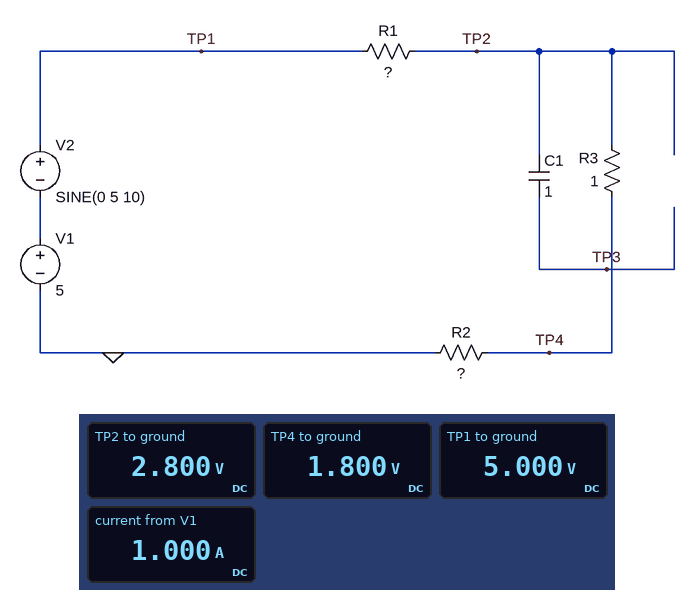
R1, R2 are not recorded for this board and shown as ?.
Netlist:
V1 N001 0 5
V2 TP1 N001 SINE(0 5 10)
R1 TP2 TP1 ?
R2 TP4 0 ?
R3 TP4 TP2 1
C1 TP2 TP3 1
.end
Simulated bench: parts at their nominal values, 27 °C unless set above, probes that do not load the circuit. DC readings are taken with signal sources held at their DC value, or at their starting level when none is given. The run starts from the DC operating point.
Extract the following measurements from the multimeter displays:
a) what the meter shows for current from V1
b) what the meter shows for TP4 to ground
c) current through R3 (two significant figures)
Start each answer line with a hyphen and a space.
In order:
- 1.000 A
- 1.800 V
- 1.0 A
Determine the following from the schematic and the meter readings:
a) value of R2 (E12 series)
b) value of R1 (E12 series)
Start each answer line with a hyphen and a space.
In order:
- 1.8 Ω
- 2.2 Ω
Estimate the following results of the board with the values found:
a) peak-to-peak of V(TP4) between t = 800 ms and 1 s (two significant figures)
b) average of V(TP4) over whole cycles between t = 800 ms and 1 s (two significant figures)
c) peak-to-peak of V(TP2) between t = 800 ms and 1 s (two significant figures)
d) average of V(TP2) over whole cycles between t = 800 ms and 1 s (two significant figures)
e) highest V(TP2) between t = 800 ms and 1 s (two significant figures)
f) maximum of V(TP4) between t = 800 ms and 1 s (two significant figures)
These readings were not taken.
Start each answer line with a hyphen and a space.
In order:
- 3.6 V
- 1.8 V
- 5.6 V
- 2.8 V
- 5.6 V
- 3.6 V
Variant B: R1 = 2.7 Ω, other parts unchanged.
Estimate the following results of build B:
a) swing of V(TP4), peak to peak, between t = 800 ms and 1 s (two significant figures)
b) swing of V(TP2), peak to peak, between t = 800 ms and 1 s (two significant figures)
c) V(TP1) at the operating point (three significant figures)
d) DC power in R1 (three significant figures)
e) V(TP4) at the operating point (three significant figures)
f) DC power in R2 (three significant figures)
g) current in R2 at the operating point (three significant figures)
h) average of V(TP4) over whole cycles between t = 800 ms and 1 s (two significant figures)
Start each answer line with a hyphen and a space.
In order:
- 3.3 V
- 5.1 V
- 5.00 V
- 2.23 W
- 1.64 V
- 1.49 W
- 909 mA
- 1.6 V
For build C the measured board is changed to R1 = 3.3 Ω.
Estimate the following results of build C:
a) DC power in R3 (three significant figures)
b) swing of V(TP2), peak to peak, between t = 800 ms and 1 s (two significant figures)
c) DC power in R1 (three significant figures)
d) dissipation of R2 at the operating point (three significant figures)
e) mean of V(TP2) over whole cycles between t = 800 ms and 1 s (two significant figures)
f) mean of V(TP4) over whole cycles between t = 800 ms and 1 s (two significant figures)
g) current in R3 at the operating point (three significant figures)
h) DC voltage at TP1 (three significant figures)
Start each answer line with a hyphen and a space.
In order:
- 672 mW
- 4.6 V
- 2.22 W
- 1.21 W
- 2.3 V
- 1.5 V
- 820 mA
- 5.00 V
